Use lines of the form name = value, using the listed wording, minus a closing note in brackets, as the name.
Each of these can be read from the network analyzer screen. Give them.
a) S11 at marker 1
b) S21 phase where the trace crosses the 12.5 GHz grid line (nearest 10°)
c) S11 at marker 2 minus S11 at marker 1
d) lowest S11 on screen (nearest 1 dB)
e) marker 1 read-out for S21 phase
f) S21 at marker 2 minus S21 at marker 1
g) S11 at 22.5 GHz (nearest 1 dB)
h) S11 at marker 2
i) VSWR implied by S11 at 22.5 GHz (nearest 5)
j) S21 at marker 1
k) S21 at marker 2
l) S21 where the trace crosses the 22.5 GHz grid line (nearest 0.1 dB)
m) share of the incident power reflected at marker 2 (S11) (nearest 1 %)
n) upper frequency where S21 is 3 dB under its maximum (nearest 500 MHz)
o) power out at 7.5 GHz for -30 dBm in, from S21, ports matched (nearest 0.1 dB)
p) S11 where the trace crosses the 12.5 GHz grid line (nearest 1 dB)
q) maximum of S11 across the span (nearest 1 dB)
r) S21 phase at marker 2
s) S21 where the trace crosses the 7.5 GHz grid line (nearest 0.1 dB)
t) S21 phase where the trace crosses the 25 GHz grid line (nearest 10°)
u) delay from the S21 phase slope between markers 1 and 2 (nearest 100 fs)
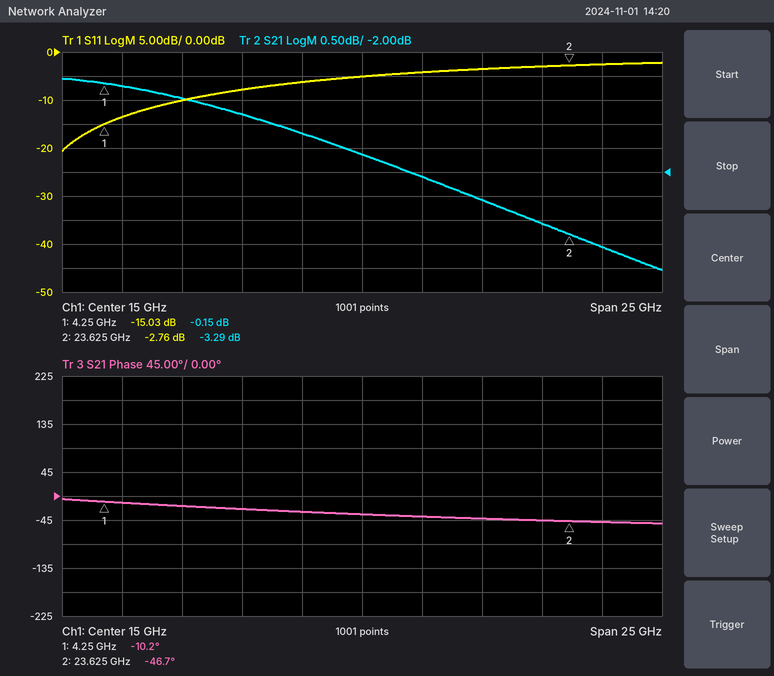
S11 at marker 1 = -15.03 dB
S21 phase where the trace crosses the 12.5 GHz grid line = -30°
S11 at marker 2 minus S11 at marker 1 = 12.27 dB
lowest S11 on screen = -21 dB
marker 1 read-out for S21 phase = -10.2°
S21 at marker 2 minus S21 at marker 1 = -3.14 dB
S11 at 22.5 GHz = -3 dB
S11 at marker 2 = -2.76 dB
VSWR implied by S11 at 22.5 GHz = 5
S21 at marker 1 = -0.15 dB
S21 at marker 2 = -3.29 dB
S21 where the trace crosses the 22.5 GHz grid line = -3.1 dB
share of the incident power reflected at marker 2 (S11) = 53 %
upper frequency where S21 is 3 dB under its maximum = 22.5 GHz
power out at 7.5 GHz for -30 dBm in, from S21, ports matched = -30.5 dBm
S11 where the trace crosses the 12.5 GHz grid line = -6 dB
maximum of S11 across the span = -2 dB
S21 phase at marker 2 = -46.7°
S21 where the trace crosses the 7.5 GHz grid line = -0.5 dB
S21 phase where the trace crosses the 25 GHz grid line = -50°
delay from the S21 phase slope between markers 1 and 2 = 5.2 ps
